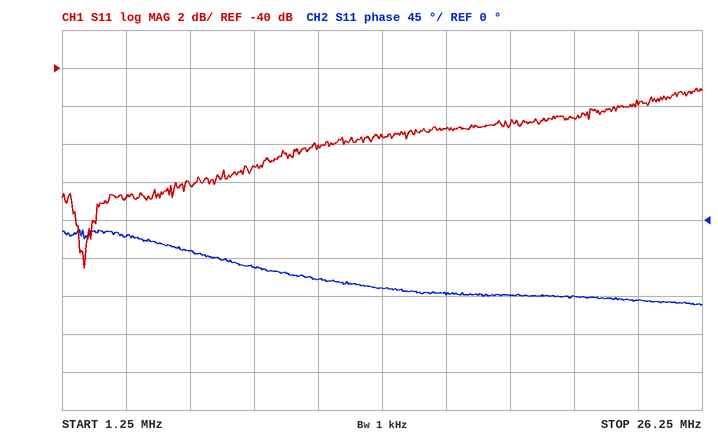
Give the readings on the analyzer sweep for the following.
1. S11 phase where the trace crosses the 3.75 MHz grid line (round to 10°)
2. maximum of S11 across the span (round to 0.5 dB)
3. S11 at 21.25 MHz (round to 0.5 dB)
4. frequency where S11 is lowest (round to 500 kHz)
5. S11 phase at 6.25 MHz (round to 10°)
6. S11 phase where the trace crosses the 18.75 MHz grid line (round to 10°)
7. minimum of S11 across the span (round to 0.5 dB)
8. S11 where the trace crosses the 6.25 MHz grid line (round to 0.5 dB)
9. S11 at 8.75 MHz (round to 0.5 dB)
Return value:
-20°
-41.0 dB
-42.5 dB
2.0 MHz
-40°
-90°
-50.5 dB
-46.0 dB
-45.0 dB
